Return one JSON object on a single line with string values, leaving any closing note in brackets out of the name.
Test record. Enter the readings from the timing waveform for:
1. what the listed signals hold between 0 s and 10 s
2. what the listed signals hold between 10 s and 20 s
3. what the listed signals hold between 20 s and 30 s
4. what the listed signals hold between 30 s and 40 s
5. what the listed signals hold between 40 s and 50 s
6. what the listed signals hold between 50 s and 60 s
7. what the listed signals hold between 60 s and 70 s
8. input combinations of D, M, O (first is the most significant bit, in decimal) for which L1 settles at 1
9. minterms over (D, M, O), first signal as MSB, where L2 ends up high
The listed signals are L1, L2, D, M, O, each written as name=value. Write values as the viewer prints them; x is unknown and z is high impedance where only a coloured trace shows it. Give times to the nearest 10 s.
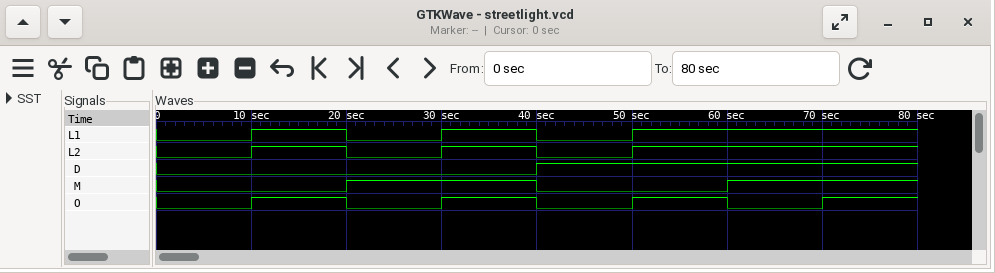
{"what the listed signals hold between 0 s and 10 s": "L1=0, L2=0, D=0, M=0, O=0", "what the listed signals hold between 10 s and 20 s": "L1=1, L2=1, D=0, M=0, O=1", "what the listed signals hold between 20 s and 30 s": "L1=0, L2=0, D=0, M=1, O=0", "what the listed signals hold between 30 s and 40 s": "L1=1, L2=1, D=0, M=1, O=1", "what the listed signals hold between 40 s and 50 s": "L1=0, L2=0, D=1, M=0, O=0", "what the listed signals hold between 50 s and 60 s": "L1=1, L2=1, D=1, M=0, O=1", "what the listed signals hold between 60 s and 70 s": "L1=1, L2=1, D=1, M=1, O=0", "input combinations of D, M, O (first is the most significant bit, in decimal) for which L1 settles at 1": "1, 3, 5, 6, 7", "minterms over (D, M, O), first signal as MSB, where L2 ends up high": "1, 3, 5, 6, 7"}
